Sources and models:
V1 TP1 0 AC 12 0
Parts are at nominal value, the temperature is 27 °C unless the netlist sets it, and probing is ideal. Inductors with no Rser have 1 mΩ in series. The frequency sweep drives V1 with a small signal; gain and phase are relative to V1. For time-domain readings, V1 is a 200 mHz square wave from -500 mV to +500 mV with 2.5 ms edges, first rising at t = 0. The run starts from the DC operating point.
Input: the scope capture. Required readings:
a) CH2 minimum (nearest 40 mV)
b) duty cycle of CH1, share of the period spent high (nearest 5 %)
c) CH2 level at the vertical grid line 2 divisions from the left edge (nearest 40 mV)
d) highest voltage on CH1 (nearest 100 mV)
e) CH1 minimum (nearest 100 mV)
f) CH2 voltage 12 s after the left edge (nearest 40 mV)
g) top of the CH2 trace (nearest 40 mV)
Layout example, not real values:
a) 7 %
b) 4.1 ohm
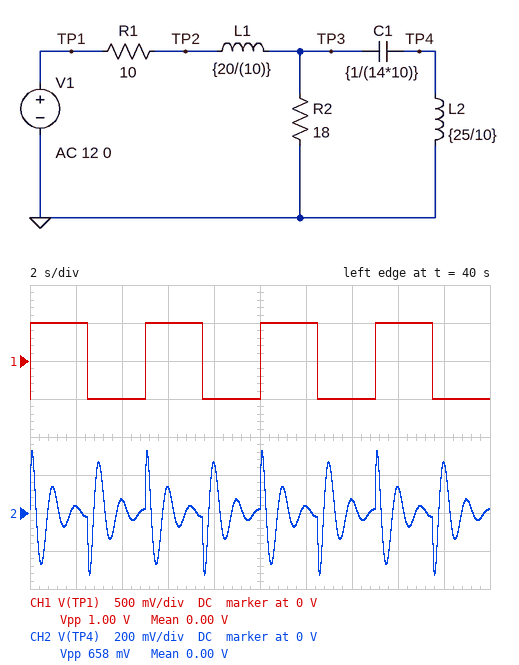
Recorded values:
a) -320 mV
b) 50 %
c) 80 mV
d) 500 mV
e) -500 mV
f) 40 mV
g) 320 mV
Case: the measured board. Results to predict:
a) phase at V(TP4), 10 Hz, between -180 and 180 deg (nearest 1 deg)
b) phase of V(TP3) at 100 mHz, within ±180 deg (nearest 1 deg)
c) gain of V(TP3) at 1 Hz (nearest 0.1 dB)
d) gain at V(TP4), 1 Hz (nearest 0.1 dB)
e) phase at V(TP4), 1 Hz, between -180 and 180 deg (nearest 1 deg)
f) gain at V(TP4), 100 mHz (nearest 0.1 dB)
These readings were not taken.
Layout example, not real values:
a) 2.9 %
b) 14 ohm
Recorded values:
a) -71 deg
b) -4 deg
c) -7.0 dB
d) 0.5 dB
e) 81 deg
f) -46.8 dB
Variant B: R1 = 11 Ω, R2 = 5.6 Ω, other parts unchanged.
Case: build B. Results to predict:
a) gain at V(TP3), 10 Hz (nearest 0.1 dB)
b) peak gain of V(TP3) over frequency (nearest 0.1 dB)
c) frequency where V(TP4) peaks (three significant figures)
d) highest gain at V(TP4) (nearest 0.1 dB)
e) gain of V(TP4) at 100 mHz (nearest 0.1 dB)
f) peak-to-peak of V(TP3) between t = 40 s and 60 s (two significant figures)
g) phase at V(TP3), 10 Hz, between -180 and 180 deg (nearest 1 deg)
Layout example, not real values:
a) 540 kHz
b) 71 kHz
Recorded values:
a) -27.1 dB
b) -9.4 dB
c) 1.17 Hz
d) 0.2 dB
e) -52.4 dB
f) 400 mV
g) -80 deg
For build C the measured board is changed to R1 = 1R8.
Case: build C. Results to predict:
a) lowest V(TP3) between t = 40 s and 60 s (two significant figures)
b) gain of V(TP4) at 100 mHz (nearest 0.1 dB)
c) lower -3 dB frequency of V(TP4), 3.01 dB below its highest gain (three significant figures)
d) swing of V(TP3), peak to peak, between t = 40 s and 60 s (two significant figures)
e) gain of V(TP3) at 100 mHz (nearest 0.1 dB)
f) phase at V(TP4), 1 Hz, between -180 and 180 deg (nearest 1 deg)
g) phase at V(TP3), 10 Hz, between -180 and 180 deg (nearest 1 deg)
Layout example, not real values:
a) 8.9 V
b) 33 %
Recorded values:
a) -680 mV
b) -43.8 dB
c) 854 mHz
d) 1.4 V
e) -0.8 dB
f) 50 deg
g) -75 deg
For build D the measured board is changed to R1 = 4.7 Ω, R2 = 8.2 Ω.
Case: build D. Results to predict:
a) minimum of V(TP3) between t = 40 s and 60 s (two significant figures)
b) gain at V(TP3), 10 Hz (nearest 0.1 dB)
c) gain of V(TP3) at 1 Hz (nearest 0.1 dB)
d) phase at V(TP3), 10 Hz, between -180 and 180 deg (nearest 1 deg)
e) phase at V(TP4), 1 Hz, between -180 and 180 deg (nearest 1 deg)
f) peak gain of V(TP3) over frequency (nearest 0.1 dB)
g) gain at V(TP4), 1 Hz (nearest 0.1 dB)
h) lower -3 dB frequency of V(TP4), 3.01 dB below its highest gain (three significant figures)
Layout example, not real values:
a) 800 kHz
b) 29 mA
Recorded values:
a) -390 mV
b) -23.8 dB
c) -7.1 dB
d) -81 deg
e) 81 deg
f) -3.9 dB
g) 0.4 dB
h) 964 mHz
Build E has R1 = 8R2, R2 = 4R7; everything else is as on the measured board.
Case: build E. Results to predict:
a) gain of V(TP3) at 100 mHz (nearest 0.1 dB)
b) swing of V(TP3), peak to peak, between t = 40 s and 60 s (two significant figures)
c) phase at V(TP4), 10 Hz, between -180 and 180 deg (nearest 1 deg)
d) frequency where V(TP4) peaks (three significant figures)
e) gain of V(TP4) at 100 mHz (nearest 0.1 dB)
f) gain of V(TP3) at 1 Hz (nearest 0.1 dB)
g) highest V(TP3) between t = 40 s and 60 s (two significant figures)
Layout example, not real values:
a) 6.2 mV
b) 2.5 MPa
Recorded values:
a) -8.8 dB
b) 420 mV
c) -82 deg
d) 1.17 Hz
e) -51.8 dB
f) -12.1 dB
g) 210 mV
